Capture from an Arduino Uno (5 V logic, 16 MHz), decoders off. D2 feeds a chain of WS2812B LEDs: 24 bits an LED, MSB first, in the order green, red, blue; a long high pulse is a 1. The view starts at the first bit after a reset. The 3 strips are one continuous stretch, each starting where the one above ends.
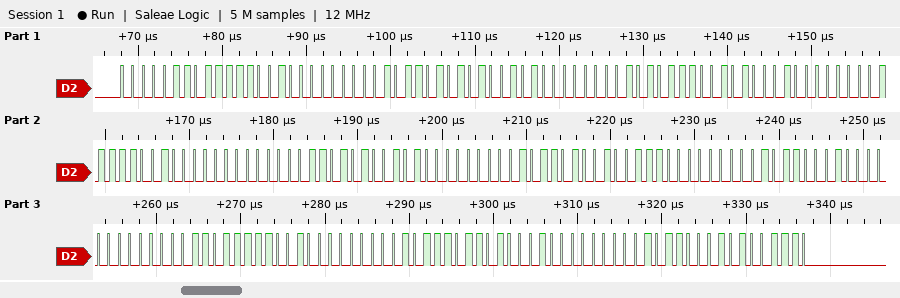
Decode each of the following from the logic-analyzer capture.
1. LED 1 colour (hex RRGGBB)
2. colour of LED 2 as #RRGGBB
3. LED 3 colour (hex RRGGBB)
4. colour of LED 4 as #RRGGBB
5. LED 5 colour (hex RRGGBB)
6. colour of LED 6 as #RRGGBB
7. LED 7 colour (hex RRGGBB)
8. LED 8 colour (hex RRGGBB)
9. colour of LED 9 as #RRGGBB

#F90600
#A55A00
#51AE00
#00F906
#00A55A
#004EB1
#0600F9
#5D00A2
#B1004E
